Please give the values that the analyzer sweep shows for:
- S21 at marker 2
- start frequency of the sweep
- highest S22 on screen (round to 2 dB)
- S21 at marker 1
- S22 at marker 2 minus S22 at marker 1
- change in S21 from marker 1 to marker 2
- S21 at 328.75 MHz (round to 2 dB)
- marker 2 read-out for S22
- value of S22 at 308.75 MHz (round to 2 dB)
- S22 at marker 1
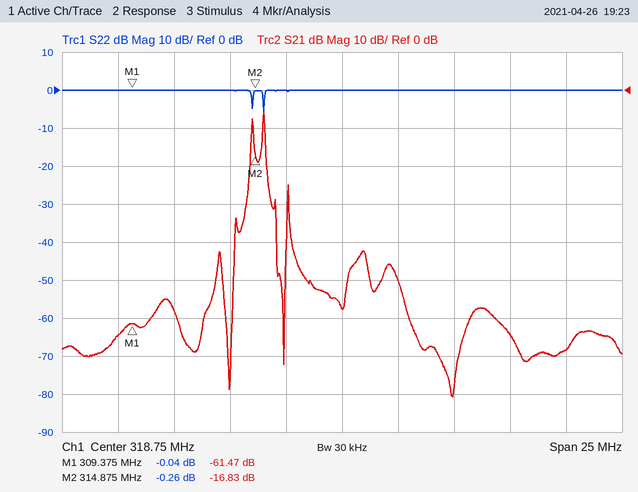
-16.83 dB
306.25 MHz
0 dB
-61.47 dB
-0.22 dB
44.64 dB
-68 dB
-0.26 dB
0 dB
-0.04 dB
